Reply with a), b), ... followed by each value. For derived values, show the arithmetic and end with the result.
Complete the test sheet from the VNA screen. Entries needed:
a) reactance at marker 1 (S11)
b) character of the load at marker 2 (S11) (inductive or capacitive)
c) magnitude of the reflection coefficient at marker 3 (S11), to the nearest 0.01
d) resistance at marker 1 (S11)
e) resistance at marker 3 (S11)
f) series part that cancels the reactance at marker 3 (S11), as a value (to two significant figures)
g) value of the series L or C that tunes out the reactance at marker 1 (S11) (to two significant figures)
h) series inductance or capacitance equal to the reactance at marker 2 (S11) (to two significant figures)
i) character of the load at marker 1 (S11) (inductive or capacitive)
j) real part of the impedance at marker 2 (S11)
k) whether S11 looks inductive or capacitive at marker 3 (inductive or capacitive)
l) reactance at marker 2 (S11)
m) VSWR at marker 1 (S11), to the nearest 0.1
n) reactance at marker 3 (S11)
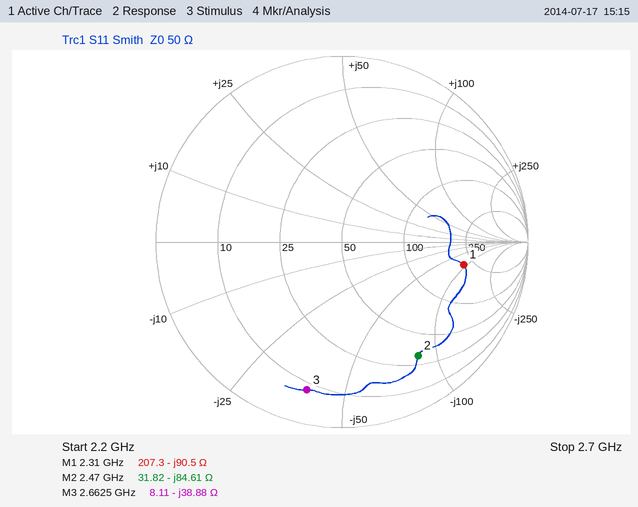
a) -90.5 Ω
b) capacitive
c) 0.82
d) 207.3 Ω
e) 8.11 Ω
f) L = 38.88 Ω/(2π × 2.6625 GHz) ≈ 2.3 nH
g) L = 90.5 Ω/(2π × 2.31 GHz) ≈ 6.2 nH
h) C = 1/(2π × 2.47 GHz × 84.61 Ω) ≈ 762 fF, so 760 fF to two significant figures
i) capacitive
j) 31.82 Ω
k) capacitive
l) -84.61 Ω
m) 5.0
n) -38.88 Ω
